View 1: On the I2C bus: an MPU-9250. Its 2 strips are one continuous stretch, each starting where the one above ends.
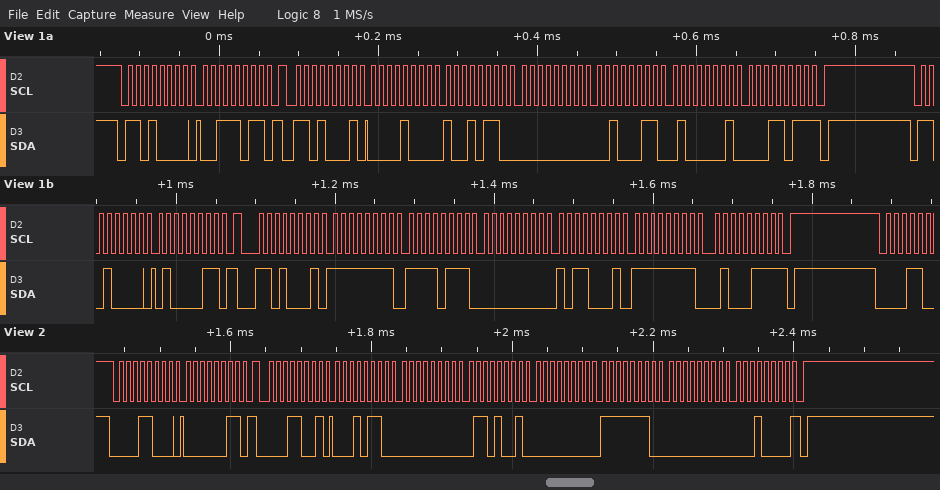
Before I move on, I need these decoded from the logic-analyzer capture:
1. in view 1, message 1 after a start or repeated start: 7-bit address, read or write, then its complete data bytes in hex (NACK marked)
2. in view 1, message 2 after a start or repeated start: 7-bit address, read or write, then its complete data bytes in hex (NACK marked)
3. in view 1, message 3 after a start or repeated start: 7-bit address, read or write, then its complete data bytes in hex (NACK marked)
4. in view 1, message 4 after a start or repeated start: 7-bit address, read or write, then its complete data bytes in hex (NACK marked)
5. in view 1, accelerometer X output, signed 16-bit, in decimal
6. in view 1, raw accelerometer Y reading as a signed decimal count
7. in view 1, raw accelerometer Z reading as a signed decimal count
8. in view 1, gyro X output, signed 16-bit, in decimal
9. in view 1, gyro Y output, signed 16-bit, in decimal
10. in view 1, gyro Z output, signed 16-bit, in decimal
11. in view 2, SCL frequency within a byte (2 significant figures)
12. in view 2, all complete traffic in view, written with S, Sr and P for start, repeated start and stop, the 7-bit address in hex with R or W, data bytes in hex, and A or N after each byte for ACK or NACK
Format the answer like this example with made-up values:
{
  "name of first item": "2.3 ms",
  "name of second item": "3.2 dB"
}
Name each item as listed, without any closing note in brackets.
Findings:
{
  "in view 1, message 1 after a start or repeated start: 7-bit address, read or write, then its complete data bytes in hex": "0x68 write: 3B",
  "in view 1, message 2 after a start or repeated start: 7-bit address, read or write, then its complete data bytes in hex": "0x68 read: 08 96 00 23 41 1B NACK",
  "in view 1, message 3 after a start or repeated start: 7-bit address, read or write, then its complete data bytes in hex": "0x68 write: 43",
  "in view 1, message 4 after a start or repeated start: 7-bit address, read or write, then its complete data bytes in hex": "0x68 read: FF F7 00 B1 FF 47 NACK",
  "in view 1, accelerometer X output, signed 16-bit, in decimal": "2198",
  "in view 1, raw accelerometer Y reading as a signed decimal count": "35",
  "in view 1, raw accelerometer Z reading as a signed decimal count": "16667",
  "in view 1, gyro X output, signed 16-bit, in decimal": "-9",
  "in view 1, gyro Y output, signed 16-bit, in decimal": "177",
  "in view 1, gyro Z output, signed 16-bit, in decimal": "-185",
  "in view 2, SCL frequency within a byte": "100 kHz",
  "in view 2, all complete traffic in view, written with S, Sr and P for start, repeated start and stop, the 7-bit address in hex with R or W, data bytes in hex, and A or N after each byte for ACK or NACK": "S 0CW A 03 A Sr 0CR A 16 A 00 A 69 A 00 A FE A 00 A 10 N P"
}
